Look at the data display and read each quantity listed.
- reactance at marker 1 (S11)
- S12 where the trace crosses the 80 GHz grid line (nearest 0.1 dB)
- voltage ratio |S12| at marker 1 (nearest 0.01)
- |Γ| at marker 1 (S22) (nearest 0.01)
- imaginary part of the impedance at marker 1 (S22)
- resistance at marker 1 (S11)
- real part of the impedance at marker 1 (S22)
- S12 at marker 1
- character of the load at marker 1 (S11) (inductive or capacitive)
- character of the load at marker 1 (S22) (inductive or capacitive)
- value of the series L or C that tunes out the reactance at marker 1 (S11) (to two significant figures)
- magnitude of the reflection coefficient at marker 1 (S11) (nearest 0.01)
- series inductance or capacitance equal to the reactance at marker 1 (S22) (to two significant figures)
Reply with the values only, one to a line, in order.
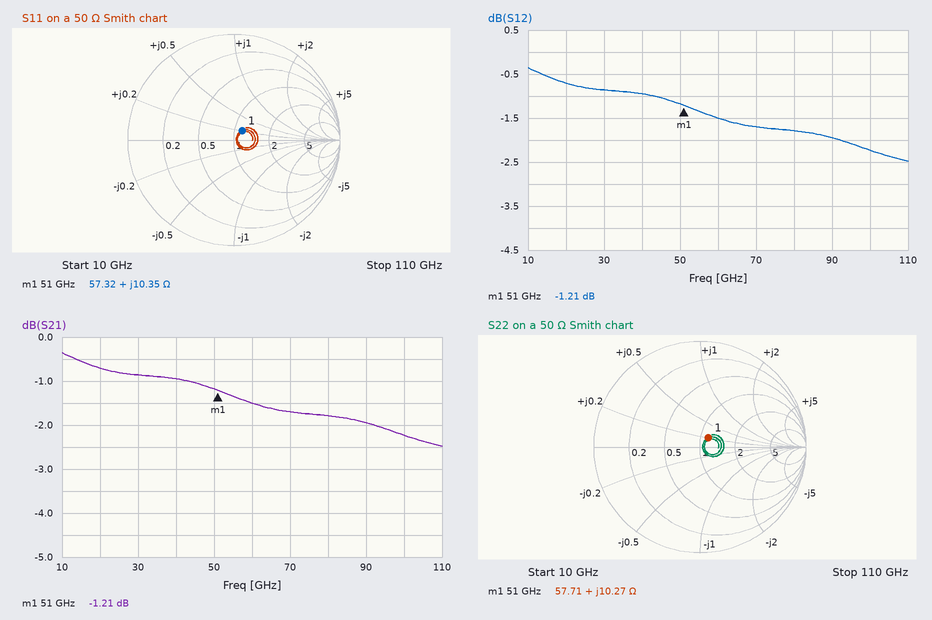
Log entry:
+10.35 Ω
-1.8 dB
0.87
0.12
+10.27 Ω
57.32 Ω
57.71 Ω
-1.21 dB
inductive
inductive
300 fF
0.12
32 pH
